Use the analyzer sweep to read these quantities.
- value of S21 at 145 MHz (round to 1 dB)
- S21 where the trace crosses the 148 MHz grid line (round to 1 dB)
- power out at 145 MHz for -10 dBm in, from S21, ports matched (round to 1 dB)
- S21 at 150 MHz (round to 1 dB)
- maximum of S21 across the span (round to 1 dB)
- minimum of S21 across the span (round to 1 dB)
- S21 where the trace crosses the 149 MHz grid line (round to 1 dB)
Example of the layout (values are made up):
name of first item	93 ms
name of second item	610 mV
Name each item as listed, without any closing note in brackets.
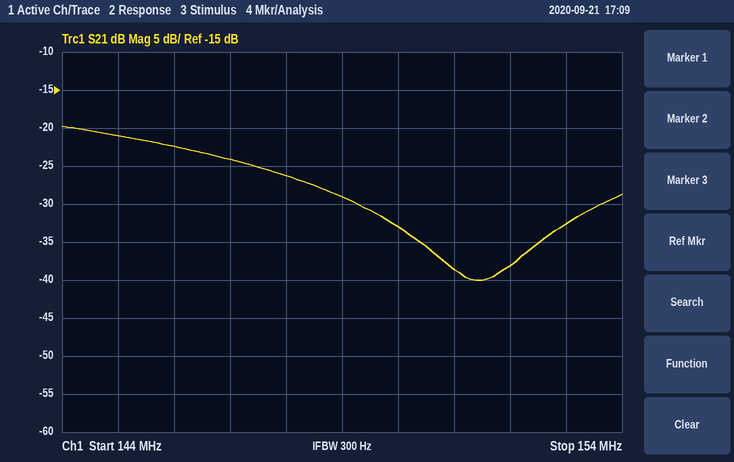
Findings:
value of S21 at 145 MHz	-21 dB
S21 where the trace crosses the 148 MHz grid line	-26 dB
power out at 145 MHz for -10 dBm in, from S21, ports matched	-31 dBm
S21 at 150 MHz	-33 dB
maximum of S21 across the span	-20 dB
minimum of S21 across the span	-40 dB
S21 where the trace crosses the 149 MHz grid line	-29 dB
